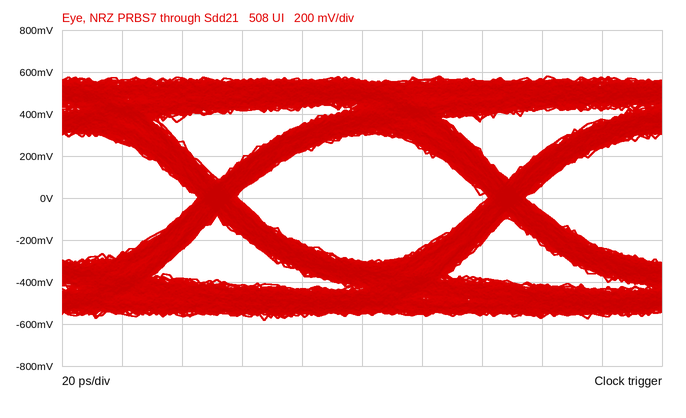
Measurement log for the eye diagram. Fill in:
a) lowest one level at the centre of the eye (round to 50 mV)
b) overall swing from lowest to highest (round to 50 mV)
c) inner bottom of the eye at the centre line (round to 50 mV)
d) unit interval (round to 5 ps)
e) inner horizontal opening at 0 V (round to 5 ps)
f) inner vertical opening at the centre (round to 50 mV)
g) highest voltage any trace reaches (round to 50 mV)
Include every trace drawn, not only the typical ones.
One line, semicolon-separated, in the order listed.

300 mV; 1.15 V; -300 mV; 95 ps; 85 ps; 600 mV; 600 mV
